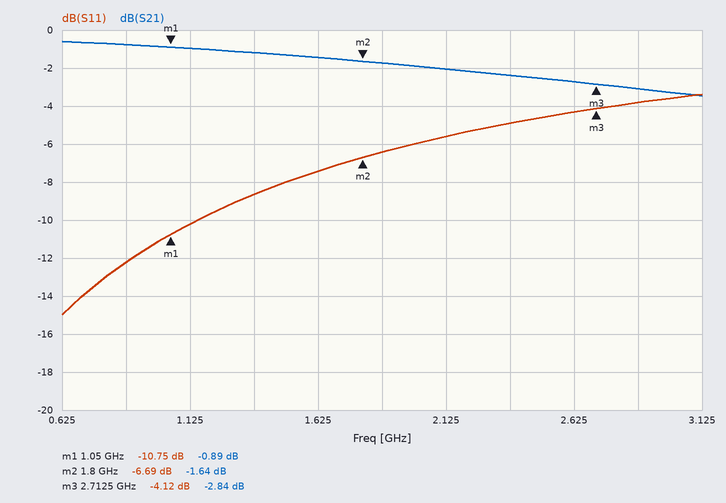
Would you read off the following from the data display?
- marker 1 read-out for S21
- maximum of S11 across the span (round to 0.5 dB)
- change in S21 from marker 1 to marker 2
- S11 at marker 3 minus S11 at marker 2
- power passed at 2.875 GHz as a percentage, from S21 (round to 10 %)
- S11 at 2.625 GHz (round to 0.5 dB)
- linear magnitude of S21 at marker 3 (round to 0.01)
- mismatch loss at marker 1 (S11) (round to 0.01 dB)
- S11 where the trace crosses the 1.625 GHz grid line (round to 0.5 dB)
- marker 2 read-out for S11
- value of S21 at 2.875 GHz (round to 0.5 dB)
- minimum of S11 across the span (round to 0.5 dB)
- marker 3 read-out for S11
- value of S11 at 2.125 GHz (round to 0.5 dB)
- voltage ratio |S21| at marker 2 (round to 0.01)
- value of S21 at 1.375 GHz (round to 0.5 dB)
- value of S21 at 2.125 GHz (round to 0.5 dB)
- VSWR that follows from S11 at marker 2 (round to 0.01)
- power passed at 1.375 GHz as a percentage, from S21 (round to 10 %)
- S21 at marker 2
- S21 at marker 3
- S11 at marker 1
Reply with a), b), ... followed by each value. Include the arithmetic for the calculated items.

a) -0.89 dB
b) -3.5 dB
c) -1.64 − (-0.89) = -0.75 dB
d) -4.12 − (-6.69) = 2.57 dB
e) 10^(-3/10) ≈ 50 %
f) -4.5 dB
g) 10^(-2.84/20) ≈ 0.72
h) −10 log10(1 − 10^(-10.75/10)) ≈ 0.38 dB
i) -7.5 dB
j) -6.69 dB
k) -3.0 dB
l) -15.0 dB
m) -4.12 dB
n) -5.5 dB
o) 10^(-1.64/20) ≈ 0.83
p) -1.0 dB
q) -2.0 dB
r) (1 + 0.4629)/(1 − 0.4629) ≈ 2.72
s) 10^(-1/10) ≈ 79.4 %, so 80 % to the nearest 10 %
t) -1.64 dB
u) -2.84 dB
v) -10.75 dB
